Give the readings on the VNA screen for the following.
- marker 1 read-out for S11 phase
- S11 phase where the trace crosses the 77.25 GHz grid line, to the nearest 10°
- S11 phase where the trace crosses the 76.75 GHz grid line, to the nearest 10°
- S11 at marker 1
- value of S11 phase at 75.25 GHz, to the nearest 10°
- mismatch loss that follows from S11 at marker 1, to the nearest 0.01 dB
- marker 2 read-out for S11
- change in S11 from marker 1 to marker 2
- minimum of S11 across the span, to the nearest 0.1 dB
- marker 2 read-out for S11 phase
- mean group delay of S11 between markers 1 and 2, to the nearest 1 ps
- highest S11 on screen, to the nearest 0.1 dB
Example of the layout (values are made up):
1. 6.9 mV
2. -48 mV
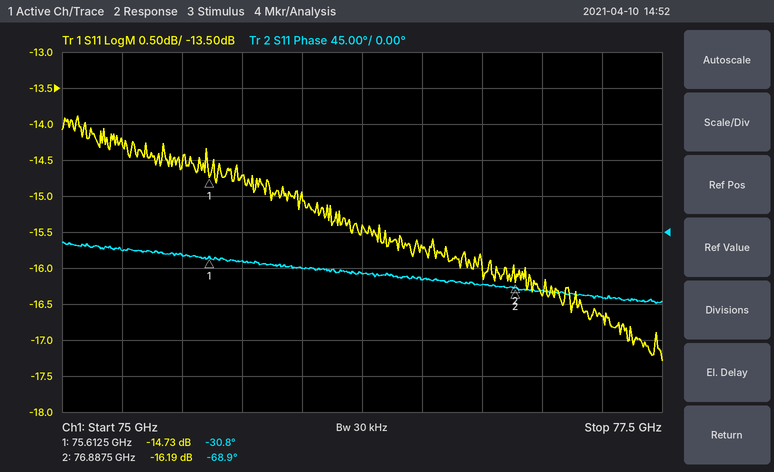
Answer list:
1. -30.8°
2. -80°
3. -70°
4. -14.73 dB
5. -20°
6. 0.15 dB
7. -16.19 dB
8. -1.46 dB
9. -17.3 dB
10. -68.9°
11. 83 ps
12. -13.9 dB
